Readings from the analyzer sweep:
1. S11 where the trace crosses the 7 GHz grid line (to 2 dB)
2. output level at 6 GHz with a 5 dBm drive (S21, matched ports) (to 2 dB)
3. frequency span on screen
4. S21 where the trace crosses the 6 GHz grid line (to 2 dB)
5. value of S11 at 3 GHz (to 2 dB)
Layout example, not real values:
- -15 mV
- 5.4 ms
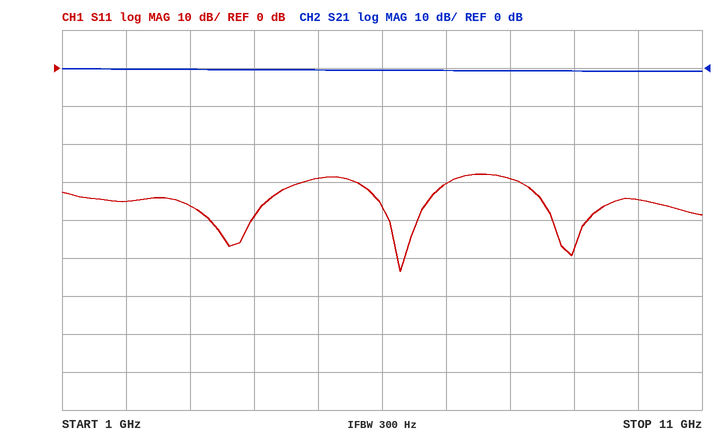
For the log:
- -30 dB
- 4 dBm
- 10 GHz
- 0 dB
- -36 dB
